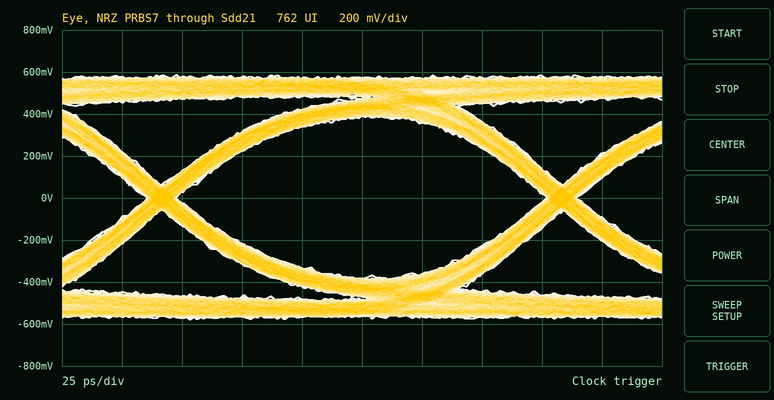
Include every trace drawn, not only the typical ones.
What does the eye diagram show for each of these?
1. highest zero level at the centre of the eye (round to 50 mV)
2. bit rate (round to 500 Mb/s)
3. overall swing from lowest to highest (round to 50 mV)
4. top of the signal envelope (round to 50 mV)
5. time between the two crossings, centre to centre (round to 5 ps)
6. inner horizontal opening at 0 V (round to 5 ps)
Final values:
-400 mV
6.0 Gb/s
1.15 V
600 mV
165 ps
155 ps
